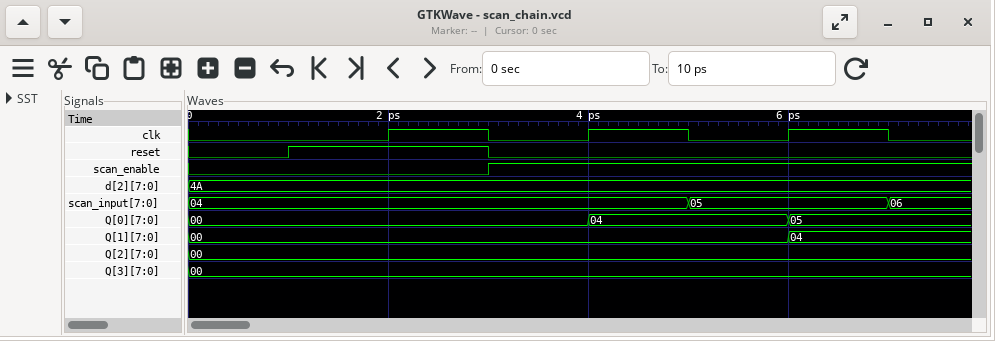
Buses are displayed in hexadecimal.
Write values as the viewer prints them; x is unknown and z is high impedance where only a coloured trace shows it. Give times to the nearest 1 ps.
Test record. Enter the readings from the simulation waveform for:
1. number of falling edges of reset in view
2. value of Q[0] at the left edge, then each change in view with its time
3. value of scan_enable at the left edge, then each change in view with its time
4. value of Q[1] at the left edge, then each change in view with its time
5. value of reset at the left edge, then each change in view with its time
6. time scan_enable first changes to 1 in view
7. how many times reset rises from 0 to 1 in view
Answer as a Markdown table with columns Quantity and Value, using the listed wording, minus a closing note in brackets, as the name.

| Quantity | Value |
|---|---|
| number of falling edges of reset in view | 1 |
| value of Q[0] at the left edge, then each change in view with its time | 00, 04 at 4 ps, 05 at 6 ps |
| value of scan_enable at the left edge, then each change in view with its time | 0, 1 at 3 ps |
| value of Q[1] at the left edge, then each change in view with its time | 00, 04 at 6 ps |
| value of reset at the left edge, then each change in view with its time | 0, 1 at 1 ps, 0 at 3 ps |
| time scan_enable first changes to 1 in view | 3 ps |
| how many times reset rises from 0 to 1 in view | 1 |
